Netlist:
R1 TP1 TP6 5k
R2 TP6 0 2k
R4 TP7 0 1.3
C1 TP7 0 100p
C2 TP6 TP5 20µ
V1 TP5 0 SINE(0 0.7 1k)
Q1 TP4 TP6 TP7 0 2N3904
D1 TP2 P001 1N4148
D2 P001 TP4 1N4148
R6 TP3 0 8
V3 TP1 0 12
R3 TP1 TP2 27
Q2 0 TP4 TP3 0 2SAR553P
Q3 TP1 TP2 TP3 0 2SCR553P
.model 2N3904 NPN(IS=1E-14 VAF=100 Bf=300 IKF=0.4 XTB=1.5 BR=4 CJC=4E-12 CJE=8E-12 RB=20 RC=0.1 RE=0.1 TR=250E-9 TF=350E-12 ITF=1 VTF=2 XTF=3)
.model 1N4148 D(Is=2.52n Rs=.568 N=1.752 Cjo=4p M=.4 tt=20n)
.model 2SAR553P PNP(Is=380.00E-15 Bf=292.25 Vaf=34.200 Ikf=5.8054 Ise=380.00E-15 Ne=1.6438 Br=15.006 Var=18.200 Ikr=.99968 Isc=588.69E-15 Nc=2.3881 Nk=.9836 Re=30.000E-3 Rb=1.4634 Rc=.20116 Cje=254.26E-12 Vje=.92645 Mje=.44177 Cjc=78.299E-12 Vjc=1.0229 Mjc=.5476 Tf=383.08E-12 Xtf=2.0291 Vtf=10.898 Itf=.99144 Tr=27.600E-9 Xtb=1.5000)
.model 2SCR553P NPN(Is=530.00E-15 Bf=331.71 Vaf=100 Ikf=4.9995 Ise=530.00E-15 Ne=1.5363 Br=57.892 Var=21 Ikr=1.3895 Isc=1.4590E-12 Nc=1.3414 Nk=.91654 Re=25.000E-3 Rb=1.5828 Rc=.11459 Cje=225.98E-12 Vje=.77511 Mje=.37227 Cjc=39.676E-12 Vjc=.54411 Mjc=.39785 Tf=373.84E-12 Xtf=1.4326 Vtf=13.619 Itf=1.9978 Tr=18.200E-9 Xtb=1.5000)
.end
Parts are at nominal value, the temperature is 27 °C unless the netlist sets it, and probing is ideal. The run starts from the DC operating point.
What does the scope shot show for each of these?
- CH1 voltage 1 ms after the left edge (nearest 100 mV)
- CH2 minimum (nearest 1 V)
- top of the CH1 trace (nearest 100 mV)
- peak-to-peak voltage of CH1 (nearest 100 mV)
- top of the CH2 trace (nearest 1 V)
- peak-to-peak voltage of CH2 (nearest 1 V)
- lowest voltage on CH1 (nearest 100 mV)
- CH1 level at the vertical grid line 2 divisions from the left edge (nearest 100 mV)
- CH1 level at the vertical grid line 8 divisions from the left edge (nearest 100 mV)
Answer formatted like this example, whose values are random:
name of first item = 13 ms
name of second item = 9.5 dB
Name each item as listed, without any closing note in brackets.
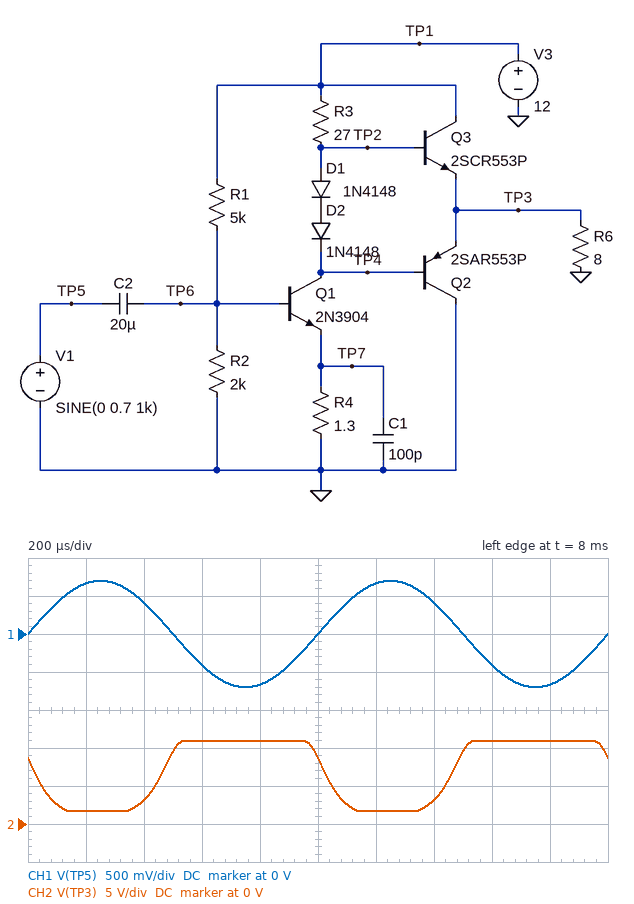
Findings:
CH1 voltage 1 ms after the left edge = 0 V
CH2 minimum = 2 V
top of the CH1 trace = 700 mV
peak-to-peak voltage of CH1 = 1.4 V
top of the CH2 trace = 11 V
peak-to-peak voltage of CH2 = 9 V
lowest voltage on CH1 = -700 mV
CH1 level at the vertical grid line 2 divisions from the left edge = 400 mV
CH1 level at the vertical grid line 8 divisions from the left edge = -400 mV
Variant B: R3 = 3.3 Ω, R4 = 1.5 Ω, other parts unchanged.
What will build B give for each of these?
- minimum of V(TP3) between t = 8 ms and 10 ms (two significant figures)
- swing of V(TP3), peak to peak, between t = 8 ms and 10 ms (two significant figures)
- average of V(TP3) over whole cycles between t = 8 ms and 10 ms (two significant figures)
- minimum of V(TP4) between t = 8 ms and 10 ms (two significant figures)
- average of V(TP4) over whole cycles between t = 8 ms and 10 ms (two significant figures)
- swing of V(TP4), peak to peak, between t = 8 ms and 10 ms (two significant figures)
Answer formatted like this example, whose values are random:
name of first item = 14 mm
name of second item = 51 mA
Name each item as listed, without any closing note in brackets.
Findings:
minimum of V(TP3) between t = 8 ms and 10 ms = 7.8 V
swing of V(TP3), peak to peak, between t = 8 ms and 10 ms = 3.4 V
average of V(TP3) over whole cycles between t = 8 ms and 10 ms = 9.7 V
minimum of V(TP4) between t = 8 ms and 10 ms = 6.8 V
average of V(TP4) over whole cycles between t = 8 ms and 10 ms = 9.1 V
swing of V(TP4), peak to peak, between t = 8 ms and 10 ms = 4.6 V
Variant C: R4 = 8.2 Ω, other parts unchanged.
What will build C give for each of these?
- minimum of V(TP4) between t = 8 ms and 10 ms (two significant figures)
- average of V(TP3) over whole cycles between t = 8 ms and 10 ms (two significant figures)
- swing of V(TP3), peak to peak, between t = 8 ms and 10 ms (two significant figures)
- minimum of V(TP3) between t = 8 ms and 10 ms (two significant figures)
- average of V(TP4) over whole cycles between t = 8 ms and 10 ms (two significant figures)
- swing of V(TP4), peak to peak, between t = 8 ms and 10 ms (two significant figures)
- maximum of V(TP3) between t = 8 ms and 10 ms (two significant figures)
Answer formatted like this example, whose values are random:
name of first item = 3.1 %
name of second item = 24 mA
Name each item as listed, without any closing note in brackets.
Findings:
minimum of V(TP4) between t = 8 ms and 10 ms = 2.7 V
average of V(TP3) over whole cycles between t = 8 ms and 10 ms = 5.7 V
swing of V(TP3), peak to peak, between t = 8 ms and 10 ms = 4.5 V
minimum of V(TP3) between t = 8 ms and 10 ms = 3.6 V
average of V(TP4) over whole cycles between t = 8 ms and 10 ms = 4.9 V
swing of V(TP4), peak to peak, between t = 8 ms and 10 ms = 4.6 V
maximum of V(TP3) between t = 8 ms and 10 ms = 8.1 V
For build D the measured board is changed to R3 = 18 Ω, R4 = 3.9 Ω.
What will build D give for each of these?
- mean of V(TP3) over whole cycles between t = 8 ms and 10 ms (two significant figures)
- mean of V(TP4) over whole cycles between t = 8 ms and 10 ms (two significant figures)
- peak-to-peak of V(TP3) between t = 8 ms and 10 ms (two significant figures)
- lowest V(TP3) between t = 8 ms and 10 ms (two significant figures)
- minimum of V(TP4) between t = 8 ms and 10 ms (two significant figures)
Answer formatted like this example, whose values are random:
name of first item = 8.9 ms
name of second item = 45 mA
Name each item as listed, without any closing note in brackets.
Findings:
mean of V(TP3) over whole cycles between t = 8 ms and 10 ms = 6.4 V
mean of V(TP4) over whole cycles between t = 8 ms and 10 ms = 5.5 V
peak-to-peak of V(TP3) between t = 8 ms and 10 ms = 6.2 V
lowest V(TP3) between t = 8 ms and 10 ms = 3.6 V
minimum of V(TP4) between t = 8 ms and 10 ms = 2.6 V
